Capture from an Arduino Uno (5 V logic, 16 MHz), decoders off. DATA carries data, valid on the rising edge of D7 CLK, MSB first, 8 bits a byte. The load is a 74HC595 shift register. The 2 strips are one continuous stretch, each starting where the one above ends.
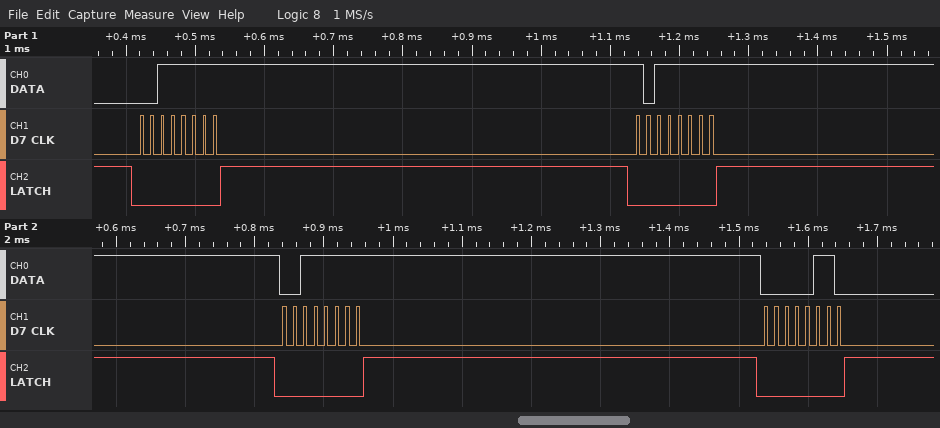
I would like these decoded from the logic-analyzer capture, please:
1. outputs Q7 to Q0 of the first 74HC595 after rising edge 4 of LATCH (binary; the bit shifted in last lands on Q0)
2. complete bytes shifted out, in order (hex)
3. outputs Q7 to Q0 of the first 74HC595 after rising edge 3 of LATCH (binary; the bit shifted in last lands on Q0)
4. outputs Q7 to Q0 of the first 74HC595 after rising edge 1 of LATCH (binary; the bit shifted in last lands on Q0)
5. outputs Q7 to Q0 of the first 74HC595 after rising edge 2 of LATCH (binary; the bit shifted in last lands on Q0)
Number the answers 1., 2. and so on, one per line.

1. 00000110
2. 3F BF 3F 06
3. 00111111
4. 00111111
5. 10111111
